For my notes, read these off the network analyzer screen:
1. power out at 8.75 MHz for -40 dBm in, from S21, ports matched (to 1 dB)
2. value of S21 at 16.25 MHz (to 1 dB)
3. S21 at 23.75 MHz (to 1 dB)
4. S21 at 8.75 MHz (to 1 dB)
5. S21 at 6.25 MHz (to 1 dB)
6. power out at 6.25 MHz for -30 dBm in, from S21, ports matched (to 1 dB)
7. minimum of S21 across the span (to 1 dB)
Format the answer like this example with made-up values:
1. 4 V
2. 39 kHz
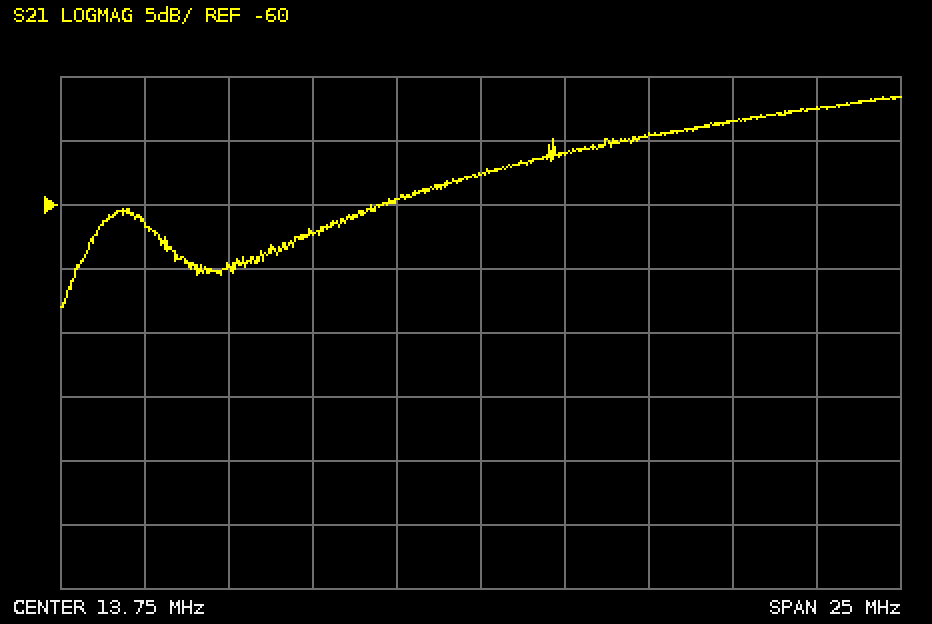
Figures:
1. -102 dBm
2. -56 dB
3. -52 dB
4. -62 dB
5. -65 dB
6. -95 dBm
7. -68 dB
